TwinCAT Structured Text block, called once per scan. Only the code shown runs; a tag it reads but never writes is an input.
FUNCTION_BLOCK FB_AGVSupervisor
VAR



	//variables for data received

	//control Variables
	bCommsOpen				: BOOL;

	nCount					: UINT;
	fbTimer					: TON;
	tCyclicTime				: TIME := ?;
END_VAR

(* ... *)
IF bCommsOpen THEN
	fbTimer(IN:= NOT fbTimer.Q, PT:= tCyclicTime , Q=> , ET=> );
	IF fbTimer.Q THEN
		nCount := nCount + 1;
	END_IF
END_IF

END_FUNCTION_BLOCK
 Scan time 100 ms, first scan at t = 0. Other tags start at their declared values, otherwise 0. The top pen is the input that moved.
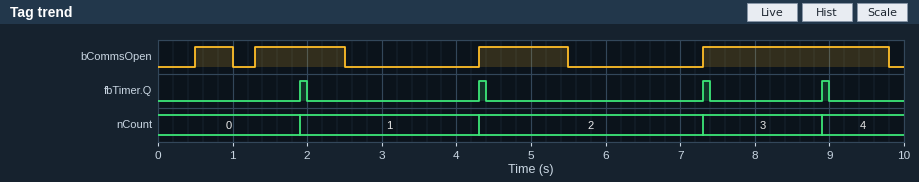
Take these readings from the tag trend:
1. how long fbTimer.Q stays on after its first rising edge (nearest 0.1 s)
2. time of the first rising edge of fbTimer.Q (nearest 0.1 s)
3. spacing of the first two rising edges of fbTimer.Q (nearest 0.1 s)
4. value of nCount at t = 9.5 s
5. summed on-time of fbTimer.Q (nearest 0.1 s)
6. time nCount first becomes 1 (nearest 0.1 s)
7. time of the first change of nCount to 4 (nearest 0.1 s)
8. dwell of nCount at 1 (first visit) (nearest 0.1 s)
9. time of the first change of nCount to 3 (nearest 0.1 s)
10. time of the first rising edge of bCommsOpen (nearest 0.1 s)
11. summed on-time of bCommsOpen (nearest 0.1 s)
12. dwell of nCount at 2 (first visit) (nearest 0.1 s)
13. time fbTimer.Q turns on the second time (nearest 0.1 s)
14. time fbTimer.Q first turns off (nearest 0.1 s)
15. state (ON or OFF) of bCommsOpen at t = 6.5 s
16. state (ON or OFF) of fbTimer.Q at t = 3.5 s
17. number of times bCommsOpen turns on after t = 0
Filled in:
0.1 s
1.9 s
2.4 s
4
0.4 s
1.9 s
8.9 s
2.4 s
7.3 s
0.5 s
5.4 s
3.0 s
4.3 s
2.0 s
OFF
OFF
4
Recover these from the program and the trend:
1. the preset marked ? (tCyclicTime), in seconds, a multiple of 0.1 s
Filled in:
1.4 s
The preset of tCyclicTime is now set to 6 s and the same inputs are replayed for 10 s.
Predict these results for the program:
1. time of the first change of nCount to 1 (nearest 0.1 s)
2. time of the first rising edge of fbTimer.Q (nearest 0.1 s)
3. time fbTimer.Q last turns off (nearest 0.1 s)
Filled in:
7.3 s
7.3 s
7.4 s
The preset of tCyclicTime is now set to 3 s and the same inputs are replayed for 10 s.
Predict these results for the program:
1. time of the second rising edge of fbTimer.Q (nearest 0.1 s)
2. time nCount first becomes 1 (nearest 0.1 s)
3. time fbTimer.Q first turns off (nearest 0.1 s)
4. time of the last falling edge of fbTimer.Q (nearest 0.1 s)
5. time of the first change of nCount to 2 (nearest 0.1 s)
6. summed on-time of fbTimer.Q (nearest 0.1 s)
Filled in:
7.5 s
4.3 s
4.4 s
7.6 s
7.5 s
0.2 s
